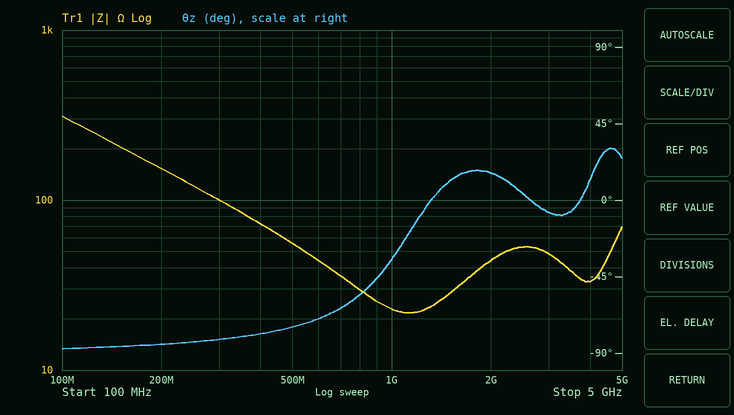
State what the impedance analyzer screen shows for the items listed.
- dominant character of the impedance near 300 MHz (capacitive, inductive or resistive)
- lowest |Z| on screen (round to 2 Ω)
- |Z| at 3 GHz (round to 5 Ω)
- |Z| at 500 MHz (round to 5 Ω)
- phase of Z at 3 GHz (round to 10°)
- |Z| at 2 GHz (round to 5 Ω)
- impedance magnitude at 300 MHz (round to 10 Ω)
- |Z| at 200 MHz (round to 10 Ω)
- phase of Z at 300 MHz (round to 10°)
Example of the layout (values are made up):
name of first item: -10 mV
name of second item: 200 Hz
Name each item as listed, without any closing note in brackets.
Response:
dominant character of the impedance near 300 MHz: capacitive
lowest |Z| on screen: 22 Ω
|Z| at 3 GHz: 50 Ω
|Z| at 500 MHz: 55 Ω
phase of Z at 3 GHz: -10°
|Z| at 2 GHz: 45 Ω
impedance magnitude at 300 MHz: 100 Ω
|Z| at 200 MHz: 150 Ω
phase of Z at 300 MHz: -80°
